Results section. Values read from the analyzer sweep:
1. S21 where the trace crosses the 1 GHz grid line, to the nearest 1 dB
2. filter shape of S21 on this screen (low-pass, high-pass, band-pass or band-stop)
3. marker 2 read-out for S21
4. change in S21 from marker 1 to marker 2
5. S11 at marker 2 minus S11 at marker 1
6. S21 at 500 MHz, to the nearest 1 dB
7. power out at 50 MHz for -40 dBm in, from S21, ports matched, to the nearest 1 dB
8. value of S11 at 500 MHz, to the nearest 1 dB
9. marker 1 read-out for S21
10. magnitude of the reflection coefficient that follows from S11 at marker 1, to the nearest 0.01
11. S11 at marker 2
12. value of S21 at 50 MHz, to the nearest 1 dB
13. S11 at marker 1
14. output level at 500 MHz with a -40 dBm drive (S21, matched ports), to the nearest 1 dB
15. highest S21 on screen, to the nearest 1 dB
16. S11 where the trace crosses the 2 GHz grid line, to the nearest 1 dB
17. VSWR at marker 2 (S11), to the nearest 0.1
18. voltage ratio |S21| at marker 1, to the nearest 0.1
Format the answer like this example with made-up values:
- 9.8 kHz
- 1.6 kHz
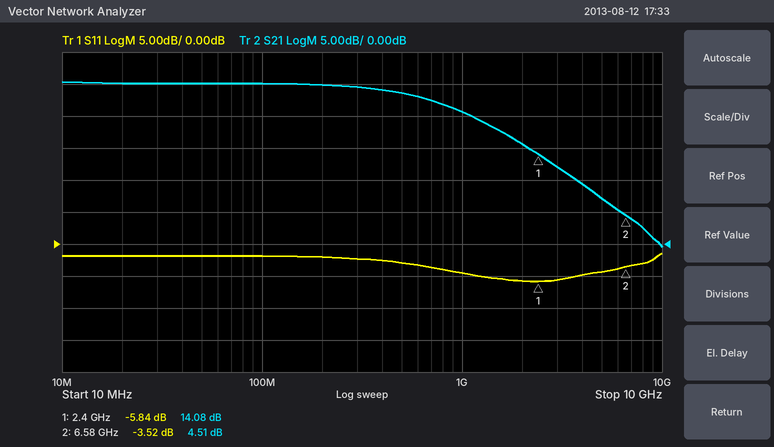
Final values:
- 21 dB
- low-pass
- 4.51 dB
- -9.57 dB
- 2.32 dB
- 24 dB
- -15 dBm
- -3 dB
- 14.08 dB
- 0.51
- -3.52 dB
- 25 dB
- -5.84 dB
- -16 dBm
- 25 dB
- -6 dB
- 5.0
- 5.1
